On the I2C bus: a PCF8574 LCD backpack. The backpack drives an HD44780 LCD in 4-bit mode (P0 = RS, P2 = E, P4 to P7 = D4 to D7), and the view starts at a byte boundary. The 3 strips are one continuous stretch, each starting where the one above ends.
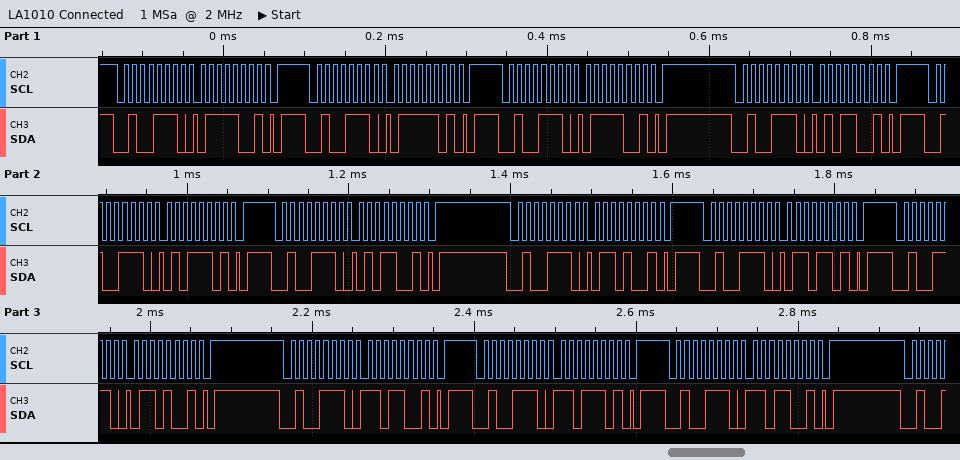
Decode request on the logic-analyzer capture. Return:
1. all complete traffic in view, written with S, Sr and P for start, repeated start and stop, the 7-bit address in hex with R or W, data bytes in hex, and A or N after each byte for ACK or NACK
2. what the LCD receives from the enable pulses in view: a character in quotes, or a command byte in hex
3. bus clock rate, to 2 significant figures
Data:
S 27W A 79 A P S 27W A 7D A P S 27W A 79 A P S 27W A 59 A P S 27W A 5D A P S 27W A 59 A P S 27W A 69 A P S 27W A 6D A P S 27W A 69 A P S 27W A D9 A P S 27W A DD A P S 27W A D9 A P
'u' 'm'
100 kHz
